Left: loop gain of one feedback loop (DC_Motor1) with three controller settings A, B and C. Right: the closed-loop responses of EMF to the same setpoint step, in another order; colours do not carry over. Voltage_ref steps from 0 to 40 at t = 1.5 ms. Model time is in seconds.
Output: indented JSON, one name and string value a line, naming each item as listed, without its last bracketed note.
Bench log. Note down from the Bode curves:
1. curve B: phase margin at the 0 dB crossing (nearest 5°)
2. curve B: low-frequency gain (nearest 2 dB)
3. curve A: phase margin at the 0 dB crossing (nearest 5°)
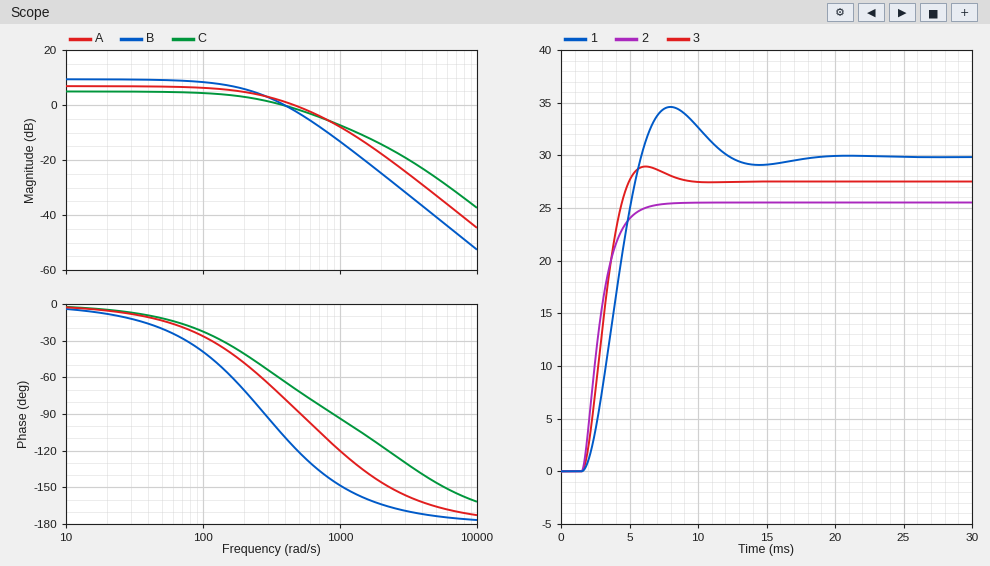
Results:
{
  "curve B: phase margin at the 0 dB crossing": "70°",
  "curve B: low-frequency gain": "10 dB",
  "curve A: phase margin at the 0 dB crossing": "95°"
}
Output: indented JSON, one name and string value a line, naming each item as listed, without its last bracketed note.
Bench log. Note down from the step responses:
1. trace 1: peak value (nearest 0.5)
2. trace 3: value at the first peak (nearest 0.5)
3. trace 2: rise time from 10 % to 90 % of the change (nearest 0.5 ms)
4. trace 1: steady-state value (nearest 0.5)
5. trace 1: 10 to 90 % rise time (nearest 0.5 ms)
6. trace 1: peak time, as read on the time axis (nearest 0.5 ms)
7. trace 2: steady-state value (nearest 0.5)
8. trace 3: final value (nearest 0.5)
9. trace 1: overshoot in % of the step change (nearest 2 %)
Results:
{
  "trace 1: peak value": "34.5",
  "trace 3: value at the first peak": "29.0",
  "trace 2: rise time from 10 % to 90 % of the change": "2.5 ms",
  "trace 1: steady-state value": "30.0",
  "trace 1: 10 to 90 % rise time": "3.0 ms",
  "trace 1: peak time, as read on the time axis": "8.0 ms",
  "trace 2: steady-state value": "25.5",
  "trace 3: final value": "27.5",
  "trace 1: overshoot in % of the step change": "16 %"
}
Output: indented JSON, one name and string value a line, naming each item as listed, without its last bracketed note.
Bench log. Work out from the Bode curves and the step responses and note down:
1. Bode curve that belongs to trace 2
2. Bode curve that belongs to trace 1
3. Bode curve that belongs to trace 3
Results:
{
  "Bode curve that belongs to trace 2": "C",
  "Bode curve that belongs to trace 1": "B",
  "Bode curve that belongs to trace 3": "A"
}
